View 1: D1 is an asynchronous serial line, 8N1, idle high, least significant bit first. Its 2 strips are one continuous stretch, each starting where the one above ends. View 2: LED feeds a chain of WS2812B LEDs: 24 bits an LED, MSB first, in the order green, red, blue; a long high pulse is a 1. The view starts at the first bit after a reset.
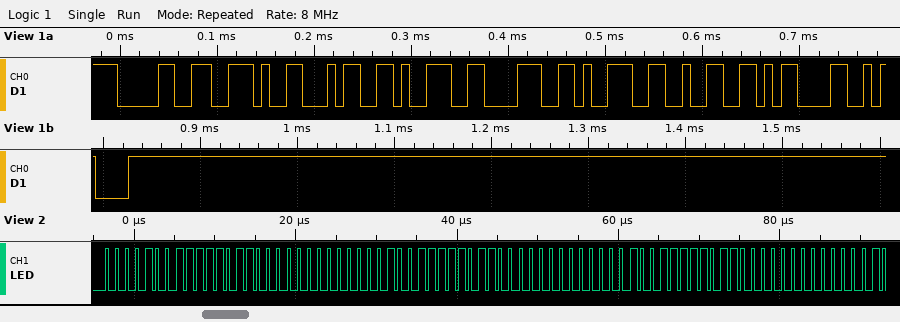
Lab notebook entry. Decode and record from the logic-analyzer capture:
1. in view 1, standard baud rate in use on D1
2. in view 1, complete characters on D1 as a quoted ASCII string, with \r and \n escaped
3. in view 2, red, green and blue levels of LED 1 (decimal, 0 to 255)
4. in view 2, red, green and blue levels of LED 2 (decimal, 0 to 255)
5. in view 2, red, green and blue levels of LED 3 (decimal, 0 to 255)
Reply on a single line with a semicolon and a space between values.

115200 baud; "0.49892\r\n"; 246, 9, 0; 246, 9, 0; 246, 9, 0
